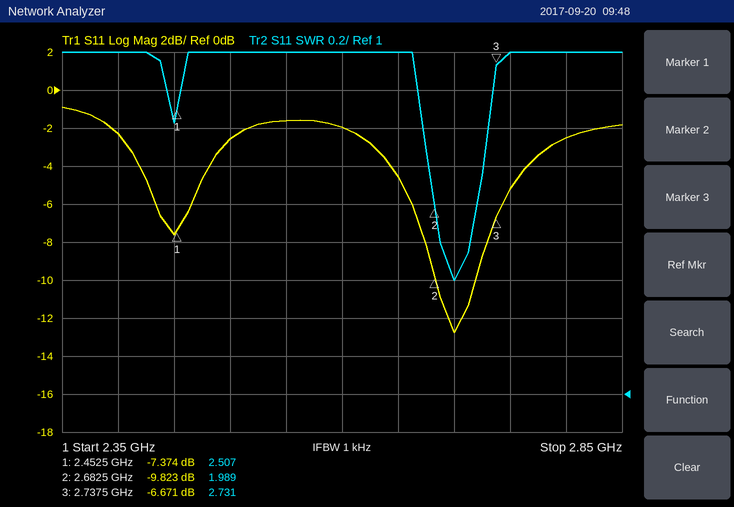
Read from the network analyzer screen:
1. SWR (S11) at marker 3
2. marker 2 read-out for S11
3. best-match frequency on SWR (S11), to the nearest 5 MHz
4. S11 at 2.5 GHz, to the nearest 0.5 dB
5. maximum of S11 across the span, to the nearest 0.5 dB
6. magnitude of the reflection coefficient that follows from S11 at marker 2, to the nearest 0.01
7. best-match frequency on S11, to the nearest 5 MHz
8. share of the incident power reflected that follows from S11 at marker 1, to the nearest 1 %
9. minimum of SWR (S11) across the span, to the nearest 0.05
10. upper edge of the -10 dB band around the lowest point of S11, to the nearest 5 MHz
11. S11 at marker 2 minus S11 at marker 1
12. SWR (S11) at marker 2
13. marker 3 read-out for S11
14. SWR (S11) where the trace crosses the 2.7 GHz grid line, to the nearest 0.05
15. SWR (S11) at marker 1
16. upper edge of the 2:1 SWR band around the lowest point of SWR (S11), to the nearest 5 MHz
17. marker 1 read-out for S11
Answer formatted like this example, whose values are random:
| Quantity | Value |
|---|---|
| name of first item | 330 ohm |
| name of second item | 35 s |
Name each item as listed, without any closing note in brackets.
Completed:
| Quantity | Value |
|---|---|
| SWR (S11) at marker 3 | 2.731 |
| marker 2 read-out for S11 | -9.823 dB |
| best-match frequency on SWR (S11), to the nearest 5 MHz | 2.700 GHz |
| S11 at 2.5 GHz, to the nearest 0.5 dB | -2.5 dB |
| maximum of S11 across the span, to the nearest 0.5 dB | -1.0 dB |
| magnitude of the reflection coefficient that follows from S11 at marker 2, to the nearest 0.01 | 0.32 |
| best-match frequency on S11, to the nearest 5 MHz | 2.700 GHz |
| share of the incident power reflected that follows from S11 at marker 1, to the nearest 1 % | 18 % |
| minimum of SWR (S11) across the span, to the nearest 0.05 | 1.60 |
| upper edge of the -10 dB band around the lowest point of S11, to the nearest 5 MHz | 2.720 GHz |
| S11 at marker 2 minus S11 at marker 1 | -2.449 dB |
| SWR (S11) at marker 2 | 1.989 |
| marker 3 read-out for S11 | -6.671 dB |
| SWR (S11) where the trace crosses the 2.7 GHz grid line, to the nearest 0.05 | 1.60 |
| SWR (S11) at marker 1 | 2.507 |
| upper edge of the 2:1 SWR band around the lowest point of SWR (S11), to the nearest 5 MHz | 2.720 GHz |
| marker 1 read-out for S11 | -7.374 dB |
